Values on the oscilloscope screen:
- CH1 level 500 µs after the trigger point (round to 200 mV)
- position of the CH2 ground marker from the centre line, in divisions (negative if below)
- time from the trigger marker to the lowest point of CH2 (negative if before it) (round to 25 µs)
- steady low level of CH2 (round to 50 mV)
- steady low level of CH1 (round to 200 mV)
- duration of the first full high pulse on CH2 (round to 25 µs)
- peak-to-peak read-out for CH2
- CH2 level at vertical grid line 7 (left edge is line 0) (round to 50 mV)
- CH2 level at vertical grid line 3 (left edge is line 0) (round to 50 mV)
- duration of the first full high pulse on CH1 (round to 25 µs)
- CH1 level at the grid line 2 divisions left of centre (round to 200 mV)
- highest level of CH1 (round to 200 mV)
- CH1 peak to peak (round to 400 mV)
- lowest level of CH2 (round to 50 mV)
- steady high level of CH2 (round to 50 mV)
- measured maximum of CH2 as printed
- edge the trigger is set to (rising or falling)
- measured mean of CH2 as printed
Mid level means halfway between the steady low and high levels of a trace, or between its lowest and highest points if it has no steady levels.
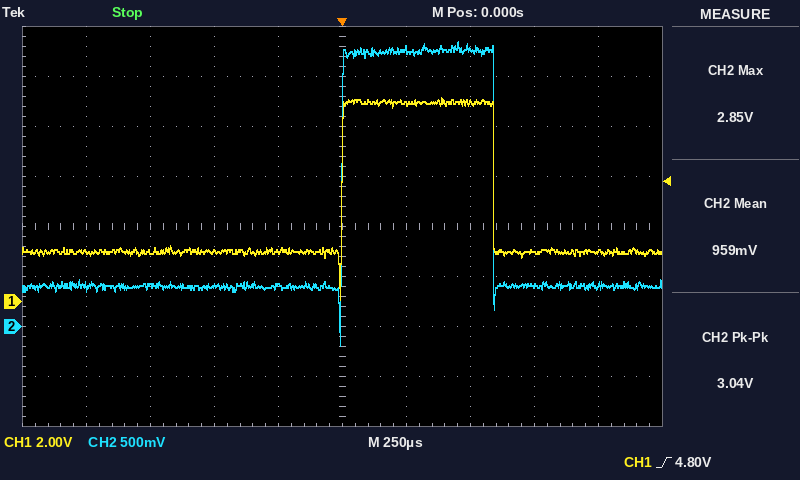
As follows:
8.0 V
-2.0 div
0 µs
400 mV
2.0 V
600 µs
3.04 V
2.80 V
400 mV
600 µs
2.0 V
8.2 V
8.0 V
-200 mV
2.75 V
2.85 V
rising
959 mV
